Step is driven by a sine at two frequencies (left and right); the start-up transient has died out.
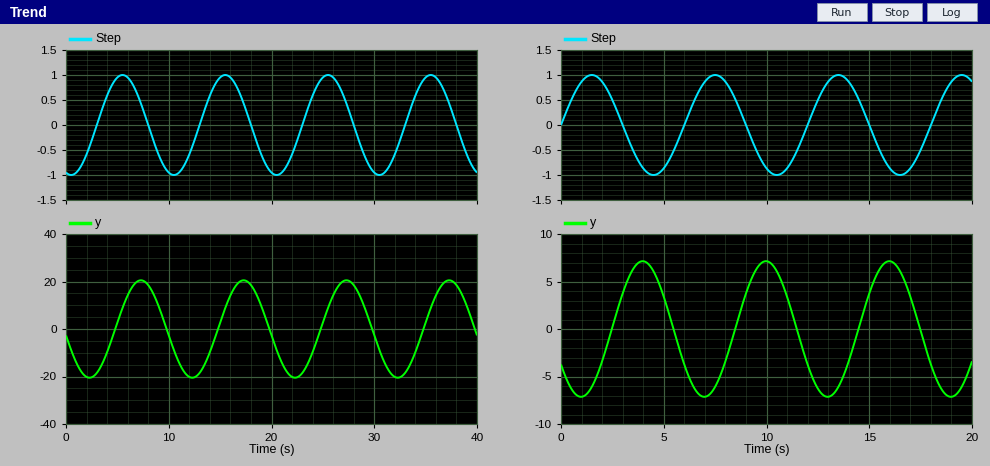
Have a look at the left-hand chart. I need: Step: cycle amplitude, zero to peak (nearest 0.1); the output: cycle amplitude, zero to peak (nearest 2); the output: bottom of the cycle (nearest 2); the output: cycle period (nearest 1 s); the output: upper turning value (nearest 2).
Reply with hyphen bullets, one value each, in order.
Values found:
- 1.0
- 20
- -20
- 10 s
- 20
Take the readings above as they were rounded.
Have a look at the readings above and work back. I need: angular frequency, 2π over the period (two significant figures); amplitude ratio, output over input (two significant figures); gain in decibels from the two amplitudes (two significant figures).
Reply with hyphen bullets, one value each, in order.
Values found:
- 0.63 rad/s
- 20
- 26 dB
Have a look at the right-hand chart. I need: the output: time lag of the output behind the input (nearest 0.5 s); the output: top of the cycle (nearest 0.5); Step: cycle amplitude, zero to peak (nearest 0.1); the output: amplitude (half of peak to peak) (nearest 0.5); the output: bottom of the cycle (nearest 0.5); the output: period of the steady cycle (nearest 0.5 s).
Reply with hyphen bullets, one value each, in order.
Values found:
- 2.5 s
- 7.0
- 1.0
- 7.0
- -7.0
- 6.0 s
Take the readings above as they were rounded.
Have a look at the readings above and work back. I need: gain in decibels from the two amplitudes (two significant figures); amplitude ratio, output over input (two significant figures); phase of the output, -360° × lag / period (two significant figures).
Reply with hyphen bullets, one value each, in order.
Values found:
- 17 dB
- 7.0
- -150°
